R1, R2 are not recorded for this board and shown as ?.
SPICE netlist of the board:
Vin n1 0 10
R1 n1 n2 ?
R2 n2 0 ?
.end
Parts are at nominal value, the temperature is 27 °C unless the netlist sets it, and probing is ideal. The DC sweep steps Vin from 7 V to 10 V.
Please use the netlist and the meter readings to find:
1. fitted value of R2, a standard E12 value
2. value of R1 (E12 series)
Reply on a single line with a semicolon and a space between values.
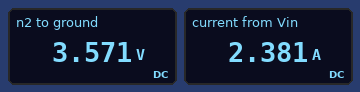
1.5 Ω; 2.7 Ω
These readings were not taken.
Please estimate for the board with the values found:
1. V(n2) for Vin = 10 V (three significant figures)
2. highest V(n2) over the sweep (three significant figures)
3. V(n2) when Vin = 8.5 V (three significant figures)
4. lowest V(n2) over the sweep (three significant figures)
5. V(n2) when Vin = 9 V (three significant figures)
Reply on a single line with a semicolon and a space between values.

3.57 V; 3.57 V; 3.04 V; 2.50 V; 3.21 V
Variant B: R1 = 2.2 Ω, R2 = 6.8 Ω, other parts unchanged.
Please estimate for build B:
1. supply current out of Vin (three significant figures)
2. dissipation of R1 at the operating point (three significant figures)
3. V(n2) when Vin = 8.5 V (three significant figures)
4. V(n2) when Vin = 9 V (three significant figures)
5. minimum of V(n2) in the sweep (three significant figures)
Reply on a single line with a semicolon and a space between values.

1.11 A; 2.72 W; 6.42 V; 6.80 V; 5.29 V
